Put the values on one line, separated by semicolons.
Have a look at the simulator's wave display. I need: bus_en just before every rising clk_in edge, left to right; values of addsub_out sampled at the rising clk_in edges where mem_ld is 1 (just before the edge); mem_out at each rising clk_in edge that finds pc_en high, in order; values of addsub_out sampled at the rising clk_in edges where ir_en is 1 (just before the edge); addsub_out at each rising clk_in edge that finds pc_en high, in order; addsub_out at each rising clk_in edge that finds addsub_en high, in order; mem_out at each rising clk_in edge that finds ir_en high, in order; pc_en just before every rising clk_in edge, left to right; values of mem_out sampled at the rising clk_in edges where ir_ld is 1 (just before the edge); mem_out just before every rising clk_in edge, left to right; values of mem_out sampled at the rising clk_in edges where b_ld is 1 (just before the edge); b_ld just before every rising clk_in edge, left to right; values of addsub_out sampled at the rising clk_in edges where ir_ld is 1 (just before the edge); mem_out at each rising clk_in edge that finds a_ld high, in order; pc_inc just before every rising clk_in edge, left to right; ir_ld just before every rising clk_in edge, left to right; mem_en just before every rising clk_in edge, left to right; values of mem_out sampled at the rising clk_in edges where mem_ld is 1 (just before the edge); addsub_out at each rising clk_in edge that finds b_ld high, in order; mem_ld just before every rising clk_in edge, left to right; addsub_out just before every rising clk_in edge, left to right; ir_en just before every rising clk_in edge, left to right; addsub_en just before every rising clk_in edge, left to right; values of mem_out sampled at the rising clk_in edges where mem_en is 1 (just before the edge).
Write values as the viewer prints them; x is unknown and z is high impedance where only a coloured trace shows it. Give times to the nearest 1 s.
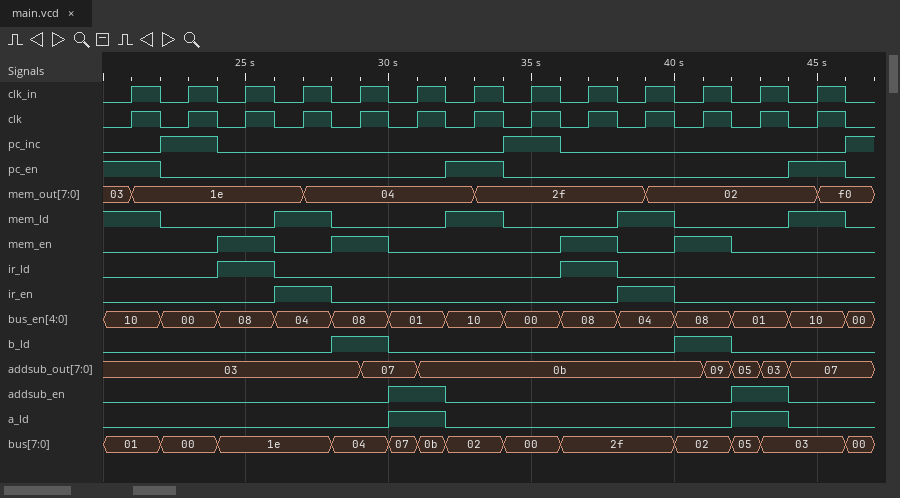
10, 00, 08, 04, 08, 01, 10, 00, 08, 04, 08, 01, 10; 03, 03, 0b, 0b, 07; 03, 04, 02; 03, 0b; 03, 0b, 07; 07, 05; 1e, 2f; 1 0 0 0 0 0 1 0 0 0 0 0 1; 1e, 2f; 03, 1e, 1e, 1e, 04, 04, 04, 2f, 2f, 2f, 02, 02, 02; 04, 02; 0 0 0 0 1 0 0 0 0 0 1 0 0; 03, 0b; 04, 02; 0 1 0 0 0 0 0 1 0 0 0 0 0; 0 0 1 0 0 0 0 0 1 0 0 0 0; 0 0 1 0 1 0 0 0 1 0 1 0 0; 03, 1e, 04, 2f, 02; 03, 0b; 1 0 0 1 0 0 1 0 0 1 0 0 1; 03, 03, 03, 03, 03, 07, 0b, 0b, 0b, 0b, 0b, 05, 07; 0 0 0 1 0 0 0 0 0 1 0 0 0; 0 0 0 0 0 1 0 0 0 0 0 1 0; 1e, 04, 2f, 02
